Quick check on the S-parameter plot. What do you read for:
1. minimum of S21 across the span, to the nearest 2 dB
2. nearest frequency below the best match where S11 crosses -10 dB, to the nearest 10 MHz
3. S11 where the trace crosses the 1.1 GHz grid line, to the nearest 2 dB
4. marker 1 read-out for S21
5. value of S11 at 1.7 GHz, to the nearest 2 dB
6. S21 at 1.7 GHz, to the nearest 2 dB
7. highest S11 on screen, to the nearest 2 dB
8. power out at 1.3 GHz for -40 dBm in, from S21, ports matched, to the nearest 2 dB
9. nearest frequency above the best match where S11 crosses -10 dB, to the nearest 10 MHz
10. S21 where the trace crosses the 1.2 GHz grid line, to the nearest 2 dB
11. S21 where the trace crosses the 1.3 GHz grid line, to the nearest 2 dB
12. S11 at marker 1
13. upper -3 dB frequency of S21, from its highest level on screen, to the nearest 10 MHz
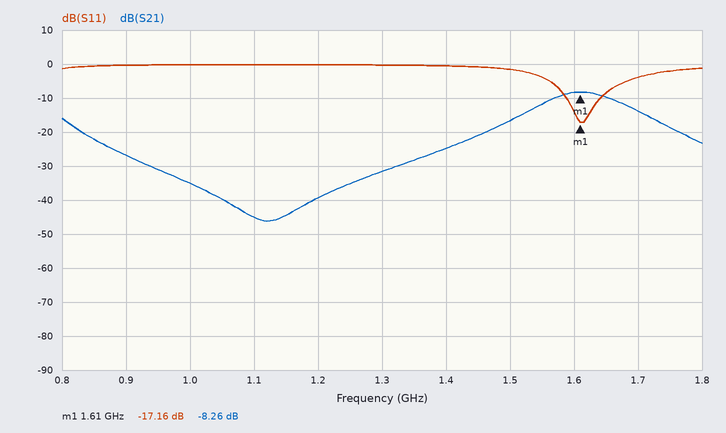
-46 dB
1.59 GHz
0 dB
-8.26 dB
-4 dB
-14 dB
0 dB
-72 dBm
1.64 GHz
-40 dB
-32 dB
-17.16 dB
1.67 GHz
